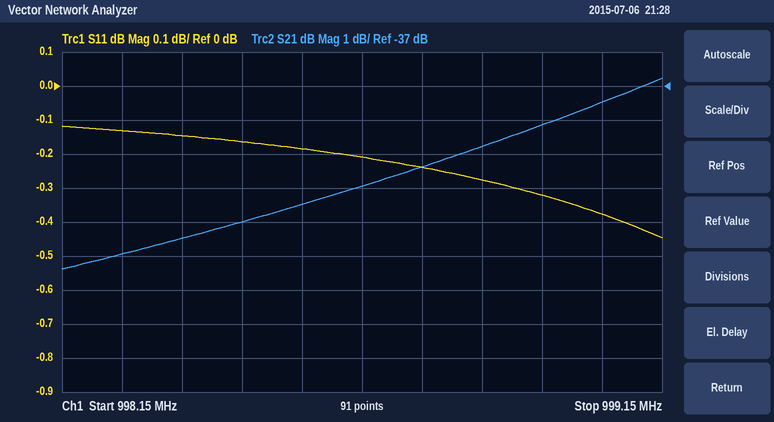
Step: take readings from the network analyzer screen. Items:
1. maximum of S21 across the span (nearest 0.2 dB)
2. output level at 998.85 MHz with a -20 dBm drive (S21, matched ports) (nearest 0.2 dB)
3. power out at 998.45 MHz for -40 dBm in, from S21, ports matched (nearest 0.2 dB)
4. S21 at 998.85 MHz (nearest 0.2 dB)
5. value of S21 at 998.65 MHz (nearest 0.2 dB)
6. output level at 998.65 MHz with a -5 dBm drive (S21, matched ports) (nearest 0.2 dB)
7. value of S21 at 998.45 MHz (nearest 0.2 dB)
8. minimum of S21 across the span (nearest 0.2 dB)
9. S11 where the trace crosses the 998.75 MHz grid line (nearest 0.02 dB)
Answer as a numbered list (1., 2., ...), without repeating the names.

1. -36.8 dB
2. -58.8 dBm
3. -81.0 dBm
4. -38.8 dB
5. -40.0 dB
6. -45.0 dBm
7. -41.0 dB
8. -42.4 dB
9. -0.24 dB
